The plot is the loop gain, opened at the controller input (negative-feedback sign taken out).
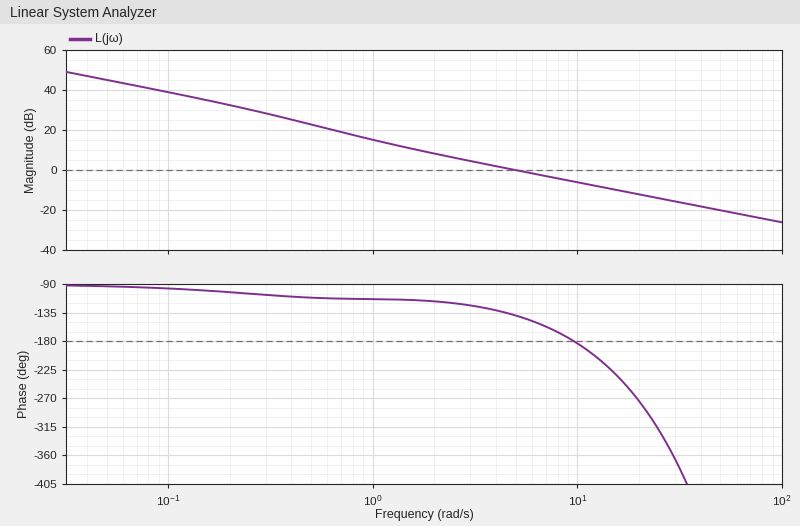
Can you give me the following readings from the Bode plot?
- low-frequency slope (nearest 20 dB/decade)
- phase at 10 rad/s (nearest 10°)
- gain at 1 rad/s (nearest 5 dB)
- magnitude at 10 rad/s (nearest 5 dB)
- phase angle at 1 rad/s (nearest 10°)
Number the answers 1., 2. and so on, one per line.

1. -20 dB/decade
2. -180°
3. 15 dB
4. -5 dB
5. -110°
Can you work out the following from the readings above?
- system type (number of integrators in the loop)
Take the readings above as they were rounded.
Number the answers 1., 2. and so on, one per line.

1. 1
